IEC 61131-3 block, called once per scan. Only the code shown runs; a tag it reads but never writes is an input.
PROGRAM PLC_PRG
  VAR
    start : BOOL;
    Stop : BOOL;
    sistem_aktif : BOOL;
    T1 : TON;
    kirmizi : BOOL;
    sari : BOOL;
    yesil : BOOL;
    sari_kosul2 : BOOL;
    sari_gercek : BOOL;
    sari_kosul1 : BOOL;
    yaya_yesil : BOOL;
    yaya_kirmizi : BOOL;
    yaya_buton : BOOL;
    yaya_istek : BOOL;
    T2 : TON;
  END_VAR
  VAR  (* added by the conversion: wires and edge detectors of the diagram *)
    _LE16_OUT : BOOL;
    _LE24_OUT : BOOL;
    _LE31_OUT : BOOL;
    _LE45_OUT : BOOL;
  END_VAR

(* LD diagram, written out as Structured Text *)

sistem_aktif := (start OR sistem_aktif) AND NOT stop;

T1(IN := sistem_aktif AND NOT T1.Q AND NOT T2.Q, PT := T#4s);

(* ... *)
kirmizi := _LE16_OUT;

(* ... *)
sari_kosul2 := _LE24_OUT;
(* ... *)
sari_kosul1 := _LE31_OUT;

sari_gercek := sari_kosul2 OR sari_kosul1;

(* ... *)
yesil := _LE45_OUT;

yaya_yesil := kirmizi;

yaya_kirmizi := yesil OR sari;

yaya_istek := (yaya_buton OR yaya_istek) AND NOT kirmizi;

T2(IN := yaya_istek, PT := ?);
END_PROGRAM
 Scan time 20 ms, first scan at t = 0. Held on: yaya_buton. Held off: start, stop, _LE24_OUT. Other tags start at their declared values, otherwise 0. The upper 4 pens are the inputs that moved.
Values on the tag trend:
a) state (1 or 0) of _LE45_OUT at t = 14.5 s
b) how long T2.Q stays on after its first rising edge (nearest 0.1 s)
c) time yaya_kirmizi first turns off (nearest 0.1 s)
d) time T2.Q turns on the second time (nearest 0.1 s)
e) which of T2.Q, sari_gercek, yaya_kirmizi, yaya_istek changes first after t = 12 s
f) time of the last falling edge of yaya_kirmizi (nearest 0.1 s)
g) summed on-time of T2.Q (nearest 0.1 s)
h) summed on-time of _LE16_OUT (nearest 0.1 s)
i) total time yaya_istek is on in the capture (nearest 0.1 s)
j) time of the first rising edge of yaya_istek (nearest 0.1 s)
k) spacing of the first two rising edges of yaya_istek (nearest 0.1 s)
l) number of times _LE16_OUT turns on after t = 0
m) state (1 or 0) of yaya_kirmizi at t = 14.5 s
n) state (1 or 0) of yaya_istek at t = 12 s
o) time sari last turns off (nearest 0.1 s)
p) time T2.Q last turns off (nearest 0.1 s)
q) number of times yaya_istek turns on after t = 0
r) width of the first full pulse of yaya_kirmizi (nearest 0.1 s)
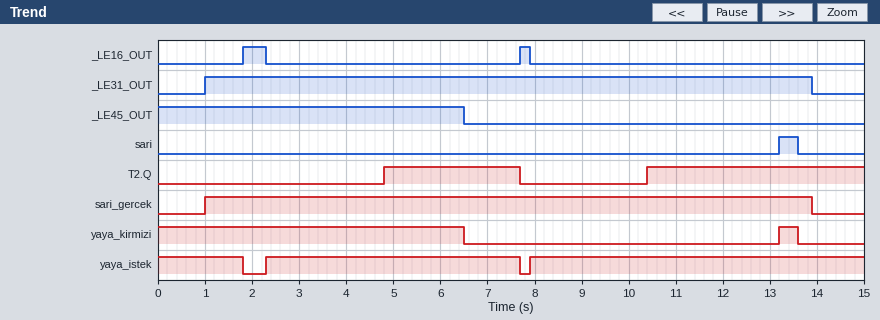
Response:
0
2.9 s
6.5 s
10.4 s
yaya_kirmizi
13.6 s
7.5 s
0.7 s
14.3 s
2.3 s
5.6 s
2
0
1
13.6 s
7.7 s
2
0.4 s
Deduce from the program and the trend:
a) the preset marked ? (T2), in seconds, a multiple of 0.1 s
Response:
2.5 s
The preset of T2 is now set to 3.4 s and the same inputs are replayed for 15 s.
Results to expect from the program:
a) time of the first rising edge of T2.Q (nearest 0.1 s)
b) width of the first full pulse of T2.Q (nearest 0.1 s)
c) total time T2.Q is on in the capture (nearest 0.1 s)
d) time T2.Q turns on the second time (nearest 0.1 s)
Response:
5.7 s
2.0 s
5.7 s
11.3 s
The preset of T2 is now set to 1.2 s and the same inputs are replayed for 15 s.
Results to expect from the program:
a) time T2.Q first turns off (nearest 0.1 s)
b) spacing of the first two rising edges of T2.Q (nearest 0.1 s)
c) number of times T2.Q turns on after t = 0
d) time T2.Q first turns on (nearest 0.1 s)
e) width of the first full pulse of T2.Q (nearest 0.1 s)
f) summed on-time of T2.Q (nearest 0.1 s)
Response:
1.8 s
2.3 s
3
1.2 s
0.6 s
10.7 s
